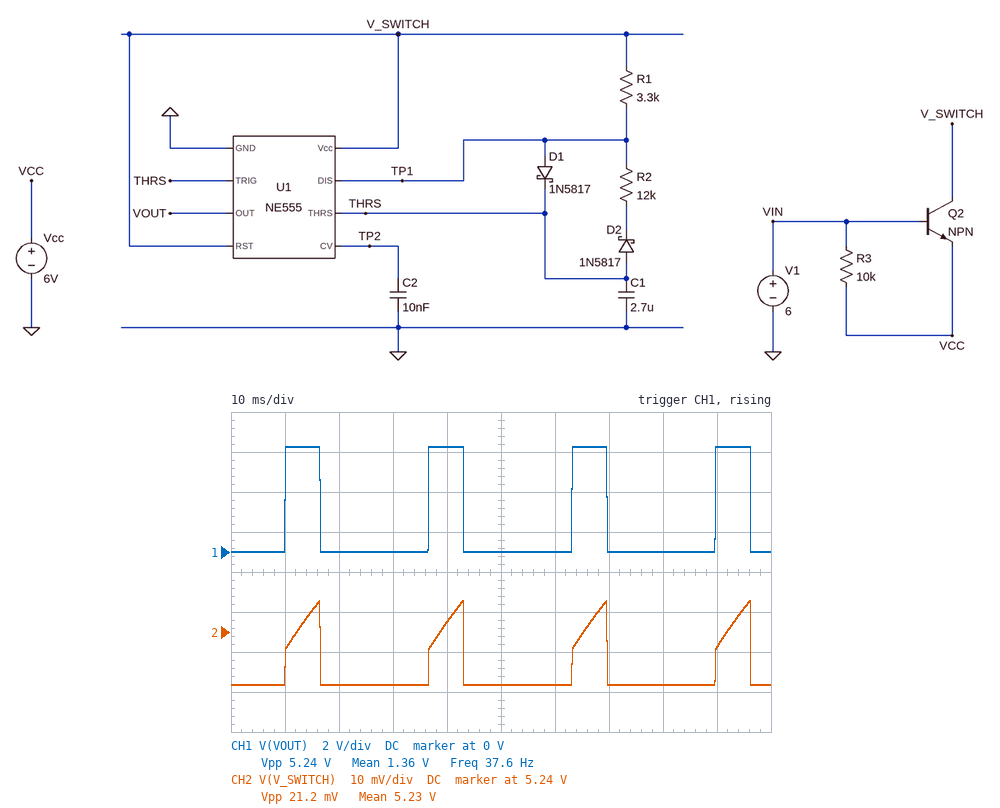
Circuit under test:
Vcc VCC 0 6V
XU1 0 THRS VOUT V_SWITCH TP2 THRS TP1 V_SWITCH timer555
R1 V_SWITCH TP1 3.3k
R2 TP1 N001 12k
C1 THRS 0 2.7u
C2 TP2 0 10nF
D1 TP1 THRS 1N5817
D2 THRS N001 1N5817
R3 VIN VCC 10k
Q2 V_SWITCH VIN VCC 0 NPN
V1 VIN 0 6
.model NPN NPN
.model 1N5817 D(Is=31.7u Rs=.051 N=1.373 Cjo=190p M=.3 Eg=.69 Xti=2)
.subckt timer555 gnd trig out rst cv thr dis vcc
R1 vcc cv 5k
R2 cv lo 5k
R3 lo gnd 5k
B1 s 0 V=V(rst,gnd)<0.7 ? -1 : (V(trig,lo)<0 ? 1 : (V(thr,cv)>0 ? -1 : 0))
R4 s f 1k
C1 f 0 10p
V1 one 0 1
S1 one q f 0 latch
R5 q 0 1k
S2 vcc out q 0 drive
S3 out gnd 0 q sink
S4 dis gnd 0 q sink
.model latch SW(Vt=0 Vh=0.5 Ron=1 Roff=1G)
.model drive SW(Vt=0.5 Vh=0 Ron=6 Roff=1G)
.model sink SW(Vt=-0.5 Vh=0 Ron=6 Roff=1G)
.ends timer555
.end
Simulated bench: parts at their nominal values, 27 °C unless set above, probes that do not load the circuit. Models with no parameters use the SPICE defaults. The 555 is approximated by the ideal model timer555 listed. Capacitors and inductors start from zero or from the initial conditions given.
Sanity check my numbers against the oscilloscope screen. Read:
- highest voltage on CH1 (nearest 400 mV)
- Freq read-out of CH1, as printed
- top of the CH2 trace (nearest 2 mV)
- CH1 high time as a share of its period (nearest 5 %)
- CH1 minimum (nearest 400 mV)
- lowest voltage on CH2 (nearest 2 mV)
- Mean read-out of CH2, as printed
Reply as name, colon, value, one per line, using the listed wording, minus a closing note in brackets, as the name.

highest voltage on CH1: 5.2 V
Freq read-out of CH1, as printed: 37.6 Hz
top of the CH2 trace: 5.248 V
CH1 high time as a share of its period: 25 %
CH1 minimum: 0 V
lowest voltage on CH2: 5.226 V
Mean read-out of CH2, as printed: 5.23 V
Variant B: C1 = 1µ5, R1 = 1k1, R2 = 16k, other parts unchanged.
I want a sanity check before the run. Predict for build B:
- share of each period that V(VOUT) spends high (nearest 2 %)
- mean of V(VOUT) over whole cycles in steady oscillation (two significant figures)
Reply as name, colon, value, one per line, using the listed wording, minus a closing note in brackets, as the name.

share of each period that V(VOUT) spends high: 8 %
mean of V(VOUT) over whole cycles in steady oscillation: 410 mV
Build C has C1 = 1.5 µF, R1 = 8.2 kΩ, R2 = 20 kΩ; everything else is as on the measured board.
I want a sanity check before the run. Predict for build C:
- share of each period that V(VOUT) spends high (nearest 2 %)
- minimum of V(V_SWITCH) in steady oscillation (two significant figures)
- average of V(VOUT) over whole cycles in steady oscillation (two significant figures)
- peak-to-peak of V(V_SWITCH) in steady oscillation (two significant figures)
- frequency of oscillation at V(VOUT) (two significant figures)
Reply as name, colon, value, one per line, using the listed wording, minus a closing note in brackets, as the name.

share of each period that V(VOUT) spends high: 34 %
minimum of V(V_SWITCH) in steady oscillation: 5.2 V
average of V(VOUT) over whole cycles in steady oscillation: 1.8 V
peak-to-peak of V(V_SWITCH) in steady oscillation: 15 mV
frequency of oscillation at V(VOUT): 39 Hz
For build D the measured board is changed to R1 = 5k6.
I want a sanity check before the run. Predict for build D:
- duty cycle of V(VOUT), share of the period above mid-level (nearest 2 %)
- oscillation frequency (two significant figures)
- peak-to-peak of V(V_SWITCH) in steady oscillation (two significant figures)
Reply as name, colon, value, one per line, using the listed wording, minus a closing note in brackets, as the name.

duty cycle of V(VOUT), share of the period above mid-level: 36 %
oscillation frequency: 32 Hz
peak-to-peak of V(V_SWITCH) in steady oscillation: 18 mV
